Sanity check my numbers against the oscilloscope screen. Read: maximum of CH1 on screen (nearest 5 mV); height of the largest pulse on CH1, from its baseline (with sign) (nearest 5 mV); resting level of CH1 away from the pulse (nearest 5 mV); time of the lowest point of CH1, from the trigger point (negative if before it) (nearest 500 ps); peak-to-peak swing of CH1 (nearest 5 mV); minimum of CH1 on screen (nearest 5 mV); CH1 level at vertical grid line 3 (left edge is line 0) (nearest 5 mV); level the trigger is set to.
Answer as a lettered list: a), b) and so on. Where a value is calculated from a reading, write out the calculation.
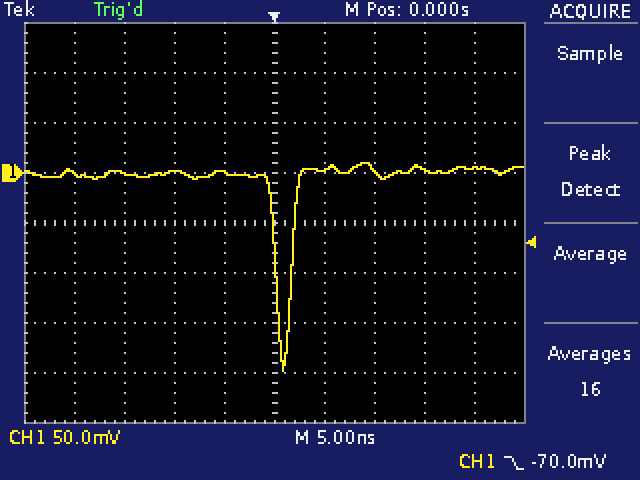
a) 10 mV
b) -200 mV − (0 mV) = -200 mV
c) 0 mV
d) +1.0 ns
e) 10 mV − (-200 mV) = 210 mV
f) -200 mV
g) 0 mV
h) -70.0 mV
